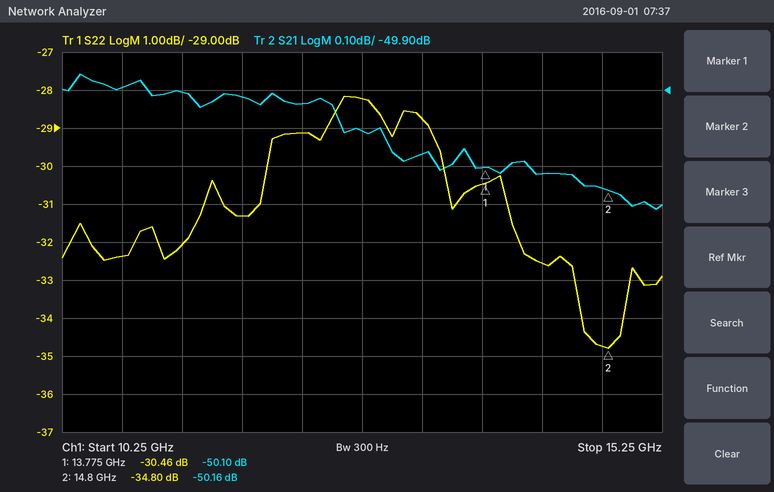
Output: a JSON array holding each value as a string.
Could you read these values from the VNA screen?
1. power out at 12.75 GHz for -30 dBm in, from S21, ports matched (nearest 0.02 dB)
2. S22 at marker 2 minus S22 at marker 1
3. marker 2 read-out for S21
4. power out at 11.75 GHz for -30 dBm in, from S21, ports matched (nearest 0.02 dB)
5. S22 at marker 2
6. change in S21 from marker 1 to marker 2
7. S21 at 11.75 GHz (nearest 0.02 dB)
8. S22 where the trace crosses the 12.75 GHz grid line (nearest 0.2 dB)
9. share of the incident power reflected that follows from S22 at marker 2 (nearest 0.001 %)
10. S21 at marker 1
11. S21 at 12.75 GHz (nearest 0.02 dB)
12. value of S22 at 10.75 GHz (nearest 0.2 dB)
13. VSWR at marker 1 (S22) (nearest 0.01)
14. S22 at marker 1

["-80.00 dBm", "-4.34 dB", "-50.16 dB", "-79.92 dBm", "-34.80 dB", "-0.06 dB", "-49.92 dB", "-28.2 dB", "0.033 %", "-50.10 dB", "-50.00 dB", "-32.4 dB", "1.06", "-30.46 dB"]
